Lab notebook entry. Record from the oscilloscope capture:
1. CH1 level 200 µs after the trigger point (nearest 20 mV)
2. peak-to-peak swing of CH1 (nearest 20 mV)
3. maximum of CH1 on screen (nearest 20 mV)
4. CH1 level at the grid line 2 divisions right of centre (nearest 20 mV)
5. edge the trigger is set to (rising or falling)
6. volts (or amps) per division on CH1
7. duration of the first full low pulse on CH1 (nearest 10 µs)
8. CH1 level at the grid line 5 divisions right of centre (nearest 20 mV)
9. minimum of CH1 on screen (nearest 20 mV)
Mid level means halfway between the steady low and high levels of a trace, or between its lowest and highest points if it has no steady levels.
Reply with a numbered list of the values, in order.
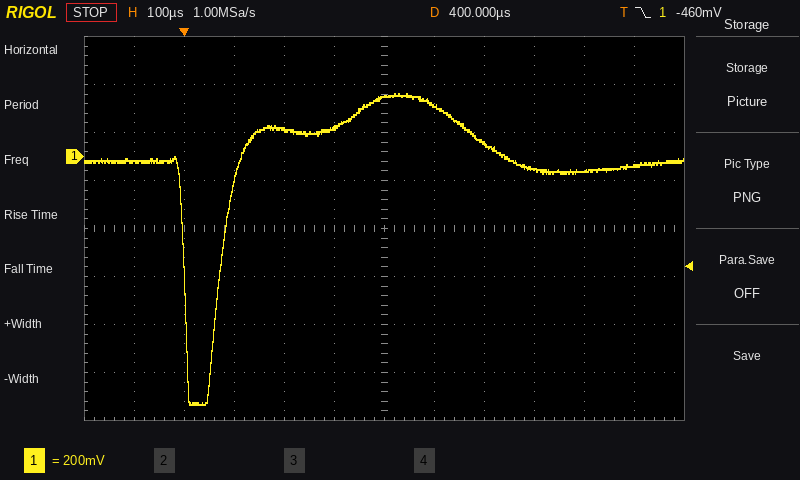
1. 120 mV
2. 1.30 V
3. 260 mV
4. 60 mV
5. falling
6. 200 mV
7. 80 µs
8. -40 mV
9. -1.04 V
